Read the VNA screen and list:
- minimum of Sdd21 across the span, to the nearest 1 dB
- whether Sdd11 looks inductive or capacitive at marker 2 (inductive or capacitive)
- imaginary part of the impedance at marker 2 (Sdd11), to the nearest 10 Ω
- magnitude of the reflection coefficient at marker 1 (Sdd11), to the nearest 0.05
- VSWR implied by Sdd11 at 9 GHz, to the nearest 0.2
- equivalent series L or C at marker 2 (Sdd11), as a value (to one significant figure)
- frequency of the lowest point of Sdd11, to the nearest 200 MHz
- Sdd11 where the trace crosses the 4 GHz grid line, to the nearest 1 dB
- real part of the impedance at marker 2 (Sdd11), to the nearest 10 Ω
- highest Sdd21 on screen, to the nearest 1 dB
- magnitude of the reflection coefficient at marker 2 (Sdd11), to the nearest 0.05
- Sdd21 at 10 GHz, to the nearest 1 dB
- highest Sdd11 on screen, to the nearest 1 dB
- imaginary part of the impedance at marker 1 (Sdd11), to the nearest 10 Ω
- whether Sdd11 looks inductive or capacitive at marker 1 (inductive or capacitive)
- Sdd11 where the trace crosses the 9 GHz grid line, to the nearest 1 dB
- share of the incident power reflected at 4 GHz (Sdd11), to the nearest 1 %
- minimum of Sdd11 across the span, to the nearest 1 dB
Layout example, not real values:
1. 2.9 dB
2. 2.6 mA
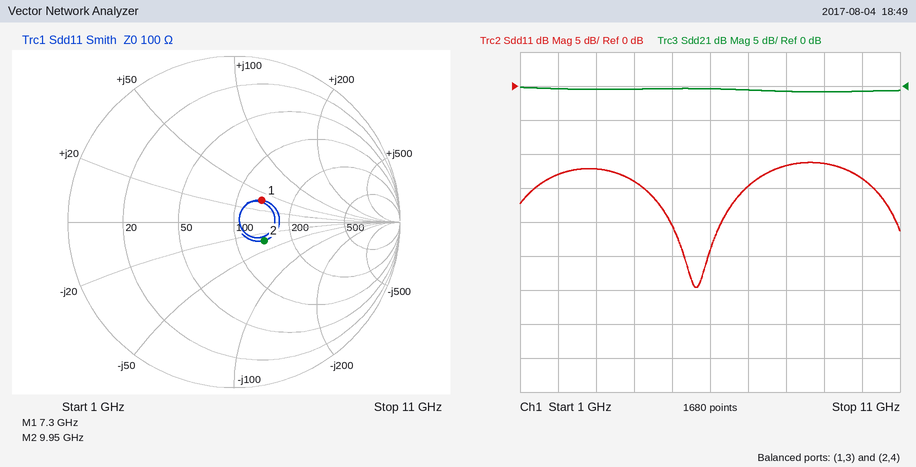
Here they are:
1. -1 dB
2. capacitive
3. -30 Ω
4. 0.20
5. 1.8
6. 500 fF
7. 5.6 GHz
8. -14 dB
9. 140 Ω
10. 0 dB
11. 0.20
12. -1 dB
13. -11 dB
14. +40 Ω
15. inductive
16. -11 dB
17. 4 %
18. -30 dB
